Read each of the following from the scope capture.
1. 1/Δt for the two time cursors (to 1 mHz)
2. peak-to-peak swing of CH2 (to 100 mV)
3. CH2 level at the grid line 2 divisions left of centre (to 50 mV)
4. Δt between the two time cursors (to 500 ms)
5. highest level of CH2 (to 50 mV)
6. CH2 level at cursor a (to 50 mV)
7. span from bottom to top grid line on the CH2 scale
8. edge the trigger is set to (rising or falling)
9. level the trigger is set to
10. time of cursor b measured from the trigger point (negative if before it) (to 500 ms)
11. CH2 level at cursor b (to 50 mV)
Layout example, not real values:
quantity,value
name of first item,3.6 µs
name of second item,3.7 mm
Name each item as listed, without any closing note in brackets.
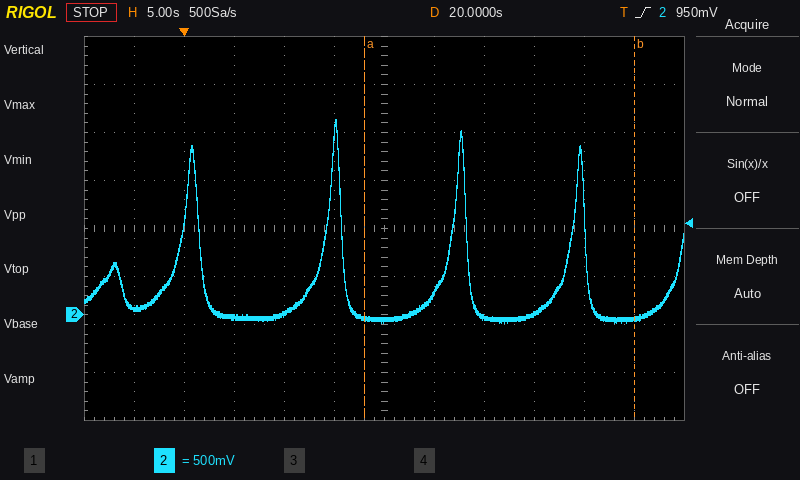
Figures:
quantity,value
1/Δt for the two time cursors,37 mHz
peak-to-peak swing of CH2,2.10 V
CH2 level at the grid line 2 divisions left of centre,0 mV
Δt between the two time cursors,27.0 s
highest level of CH2,2.05 V
CH2 level at cursor a,-50 mV
span from bottom to top grid line on the CH2 scale,4 V
edge the trigger is set to,rising
level the trigger is set to,950 mV
time of cursor b measured from the trigger point (negative if before it),+45.0 s
CH2 level at cursor b,-50 mV
